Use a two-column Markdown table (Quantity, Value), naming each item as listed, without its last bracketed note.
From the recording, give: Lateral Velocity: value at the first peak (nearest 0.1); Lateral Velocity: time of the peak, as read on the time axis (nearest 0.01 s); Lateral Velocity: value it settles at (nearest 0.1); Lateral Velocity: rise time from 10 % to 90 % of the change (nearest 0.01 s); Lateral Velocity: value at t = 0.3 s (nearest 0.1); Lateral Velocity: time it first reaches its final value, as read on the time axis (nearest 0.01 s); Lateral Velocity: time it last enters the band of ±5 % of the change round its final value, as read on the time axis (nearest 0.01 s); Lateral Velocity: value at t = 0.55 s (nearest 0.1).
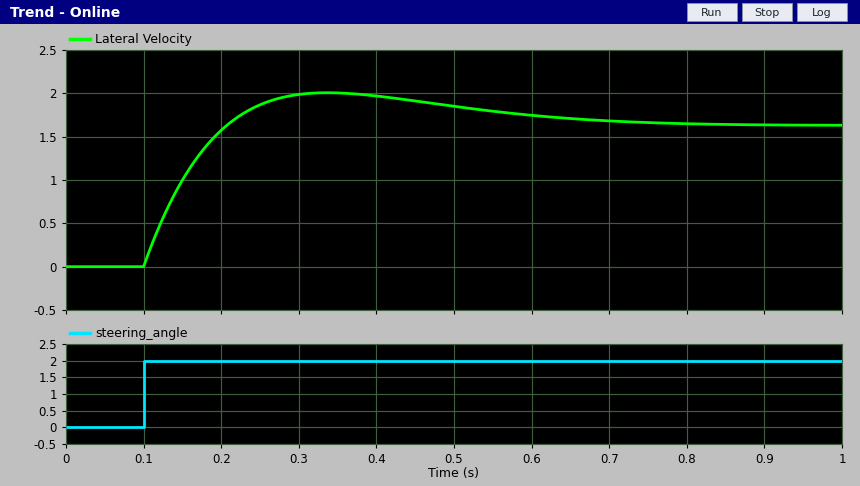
| Quantity | Value |
|---|---|
| Lateral Velocity: value at the first peak | 2.0 |
| Lateral Velocity: time of the peak, as read on the time axis | 0.34 s |
| Lateral Velocity: value it settles at | 1.6 |
| Lateral Velocity: rise time from 10 % to 90 % of the change | 0.08 s |
| Lateral Velocity: value at t = 0.3 s | 2.0 |
| Lateral Velocity: time it first reaches its final value, as read on the time axis | 0.21 s |
| Lateral Velocity: time it last enters the band of ±5 % of the change round its final value, as read on the time axis | 0.64 s |
| Lateral Velocity: value at t = 0.55 s | 1.8 |
